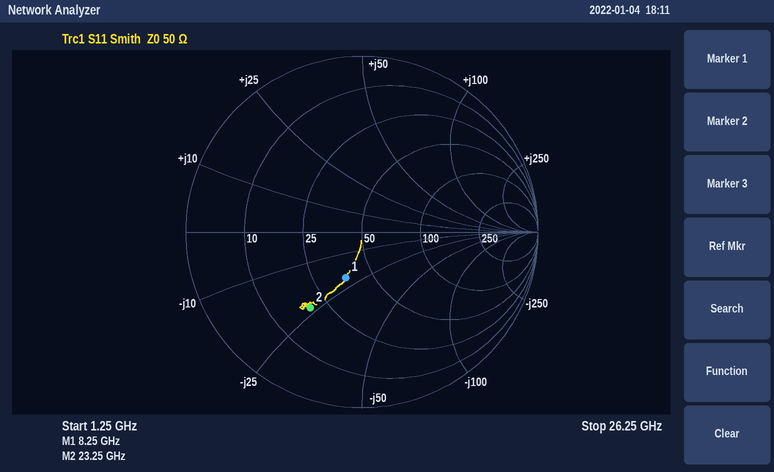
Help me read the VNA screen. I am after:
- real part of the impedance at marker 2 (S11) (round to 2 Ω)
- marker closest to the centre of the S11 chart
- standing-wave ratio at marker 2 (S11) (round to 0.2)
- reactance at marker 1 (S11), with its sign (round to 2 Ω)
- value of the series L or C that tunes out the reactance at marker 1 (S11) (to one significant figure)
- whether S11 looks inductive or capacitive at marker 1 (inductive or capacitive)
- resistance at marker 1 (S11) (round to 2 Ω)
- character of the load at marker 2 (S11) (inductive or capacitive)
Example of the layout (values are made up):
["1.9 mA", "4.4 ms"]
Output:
["20 Ω", "marker 1", "3.2", "-20 Ω", "400 pH", "capacitive", "36 Ω", "capacitive"]
